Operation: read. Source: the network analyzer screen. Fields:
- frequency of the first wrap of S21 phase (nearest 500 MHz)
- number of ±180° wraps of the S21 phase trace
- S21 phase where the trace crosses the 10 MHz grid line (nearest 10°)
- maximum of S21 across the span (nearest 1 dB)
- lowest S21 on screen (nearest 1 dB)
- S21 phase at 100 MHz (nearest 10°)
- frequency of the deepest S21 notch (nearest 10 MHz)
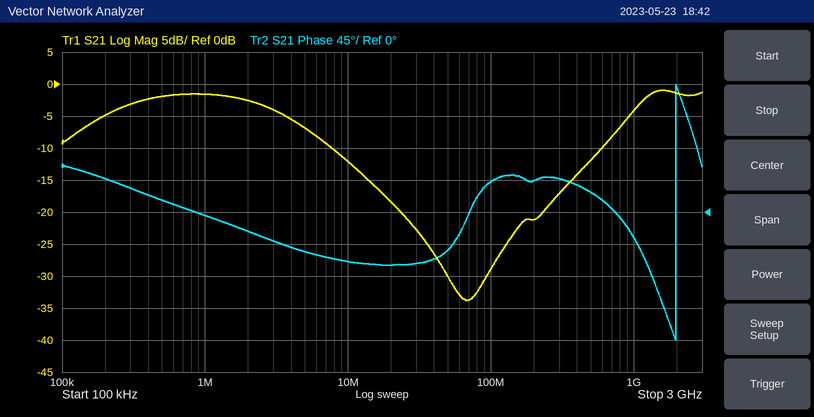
2.0 GHz
1
-70°
-1 dB
-34 dB
40°
70 MHz
